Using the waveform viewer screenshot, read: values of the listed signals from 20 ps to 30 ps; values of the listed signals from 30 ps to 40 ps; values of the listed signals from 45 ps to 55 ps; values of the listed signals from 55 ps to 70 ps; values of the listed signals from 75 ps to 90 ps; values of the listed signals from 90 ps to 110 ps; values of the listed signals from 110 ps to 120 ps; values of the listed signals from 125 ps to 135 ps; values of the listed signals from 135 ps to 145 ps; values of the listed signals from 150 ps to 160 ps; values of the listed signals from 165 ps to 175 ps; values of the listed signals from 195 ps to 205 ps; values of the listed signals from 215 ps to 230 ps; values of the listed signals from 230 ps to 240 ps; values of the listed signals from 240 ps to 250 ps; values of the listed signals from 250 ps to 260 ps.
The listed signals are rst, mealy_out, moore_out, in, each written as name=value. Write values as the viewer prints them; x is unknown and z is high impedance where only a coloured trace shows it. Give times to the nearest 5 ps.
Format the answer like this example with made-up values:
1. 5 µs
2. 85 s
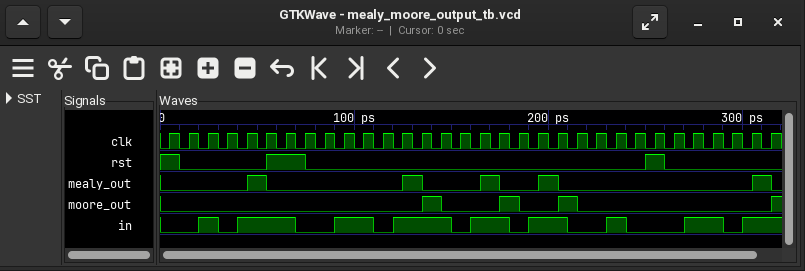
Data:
1. rst=0, mealy_out=0, moore_out=0, in=1
2. rst=0, mealy_out=0, moore_out=0, in=0
3. rst=0, mealy_out=1, moore_out=0, in=1
4. rst=1, mealy_out=0, moore_out=0, in=1
5. rst=0, mealy_out=0, moore_out=0, in=0
6. rst=0, mealy_out=0, moore_out=0, in=1
7. rst=0, mealy_out=0, moore_out=0, in=0
8. rst=0, mealy_out=1, moore_out=0, in=1
9. rst=0, mealy_out=0, moore_out=1, in=1
10. rst=0, mealy_out=0, moore_out=0, in=0
11. rst=0, mealy_out=1, moore_out=0, in=1
12. rst=0, mealy_out=1, moore_out=0, in=1
13. rst=0, mealy_out=0, moore_out=0, in=0
14. rst=0, mealy_out=0, moore_out=0, in=1
15. rst=0, mealy_out=0, moore_out=0, in=0
16. rst=1, mealy_out=0, moore_out=0, in=0
